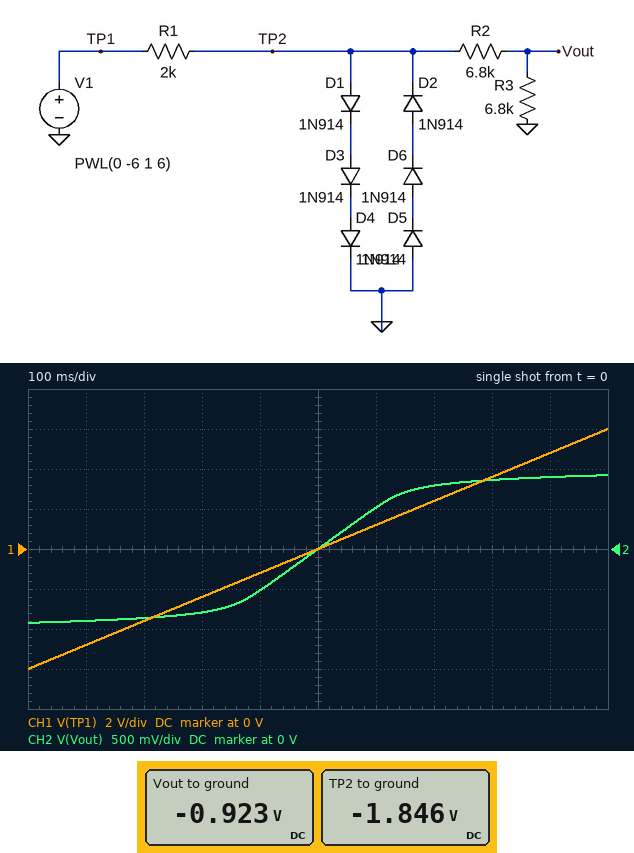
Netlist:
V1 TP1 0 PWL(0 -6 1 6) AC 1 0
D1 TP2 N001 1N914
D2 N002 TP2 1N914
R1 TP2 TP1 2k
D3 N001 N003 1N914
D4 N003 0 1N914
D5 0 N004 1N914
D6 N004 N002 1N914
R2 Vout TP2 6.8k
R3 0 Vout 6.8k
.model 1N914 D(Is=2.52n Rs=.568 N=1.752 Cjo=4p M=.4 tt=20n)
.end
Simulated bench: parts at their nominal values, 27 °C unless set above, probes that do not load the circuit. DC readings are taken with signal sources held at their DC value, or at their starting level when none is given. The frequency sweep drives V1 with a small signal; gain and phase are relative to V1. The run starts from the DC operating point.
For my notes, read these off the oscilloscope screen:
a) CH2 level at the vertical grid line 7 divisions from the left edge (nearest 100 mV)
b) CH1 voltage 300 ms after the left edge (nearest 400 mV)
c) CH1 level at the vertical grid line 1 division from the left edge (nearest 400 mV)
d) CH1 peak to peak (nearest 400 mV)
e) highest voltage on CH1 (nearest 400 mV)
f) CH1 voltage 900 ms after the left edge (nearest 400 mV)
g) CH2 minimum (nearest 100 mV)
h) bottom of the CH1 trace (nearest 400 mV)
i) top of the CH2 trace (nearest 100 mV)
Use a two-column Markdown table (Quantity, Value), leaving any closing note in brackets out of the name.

| Quantity | Value |
|---|---|
| CH2 level at the vertical grid line 7 divisions from the left edge | 800 mV |
| CH1 voltage 300 ms after the left edge | -2.4 V |
| CH1 level at the vertical grid line 1 division from the left edge | -4.8 V |
| CH1 peak to peak | 12.0 V |
| highest voltage on CH1 | 6.0 V |
| CH1 voltage 900 ms after the left edge | 4.8 V |
| CH2 minimum | -900 mV |
| bottom of the CH1 trace | -6.0 V |
| top of the CH2 trace | 900 mV |
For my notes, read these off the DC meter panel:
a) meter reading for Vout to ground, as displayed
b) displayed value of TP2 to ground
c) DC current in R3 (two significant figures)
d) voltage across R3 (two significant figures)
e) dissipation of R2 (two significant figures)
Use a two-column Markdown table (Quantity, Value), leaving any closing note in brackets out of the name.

| Quantity | Value |
|---|---|
| meter reading for Vout to ground, as displayed | -0.923 V |
| displayed value of TP2 to ground | -1.846 V |
| DC current in R3 | 140 µA |
| voltage across R3 | 920 mV |
| dissipation of R2 | 130 µW |
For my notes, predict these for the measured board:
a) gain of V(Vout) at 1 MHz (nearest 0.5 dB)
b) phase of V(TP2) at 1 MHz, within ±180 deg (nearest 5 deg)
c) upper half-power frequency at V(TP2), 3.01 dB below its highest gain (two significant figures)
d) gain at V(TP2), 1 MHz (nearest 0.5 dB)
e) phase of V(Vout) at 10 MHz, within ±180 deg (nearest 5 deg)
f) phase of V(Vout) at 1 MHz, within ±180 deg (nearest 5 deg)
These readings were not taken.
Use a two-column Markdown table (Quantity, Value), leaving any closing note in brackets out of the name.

| Quantity | Value |
|---|---|
| gain of V(Vout) at 1 MHz | -35.5 dB |
| phase of V(TP2) at 1 MHz, within ±180 deg | -5 deg |
| upper half-power frequency at V(TP2), 3.01 dB below its highest gain | 8.2 MHz |
| gain at V(TP2), 1 MHz | -29.5 dB |
| phase of V(Vout) at 10 MHz, within ±180 deg | -50 deg |
| phase of V(Vout) at 1 MHz, within ±180 deg | -5 deg |
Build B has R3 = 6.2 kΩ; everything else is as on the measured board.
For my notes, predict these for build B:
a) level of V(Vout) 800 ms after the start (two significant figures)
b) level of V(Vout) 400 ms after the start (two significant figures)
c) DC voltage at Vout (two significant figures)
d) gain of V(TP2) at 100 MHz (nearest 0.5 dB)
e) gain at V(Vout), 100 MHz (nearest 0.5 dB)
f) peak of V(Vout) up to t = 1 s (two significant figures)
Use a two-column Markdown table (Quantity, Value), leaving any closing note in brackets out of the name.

| Quantity | Value |
|---|---|
| level of V(Vout) 800 ms after the start | 820 mV |
| level of V(Vout) 400 ms after the start | -490 mV |
| DC voltage at Vout | -880 mV |
| gain of V(TP2) at 100 MHz | -50.5 dB |
| gain at V(Vout), 100 MHz | -57.0 dB |
| peak of V(Vout) up to t = 1 s | 880 mV |
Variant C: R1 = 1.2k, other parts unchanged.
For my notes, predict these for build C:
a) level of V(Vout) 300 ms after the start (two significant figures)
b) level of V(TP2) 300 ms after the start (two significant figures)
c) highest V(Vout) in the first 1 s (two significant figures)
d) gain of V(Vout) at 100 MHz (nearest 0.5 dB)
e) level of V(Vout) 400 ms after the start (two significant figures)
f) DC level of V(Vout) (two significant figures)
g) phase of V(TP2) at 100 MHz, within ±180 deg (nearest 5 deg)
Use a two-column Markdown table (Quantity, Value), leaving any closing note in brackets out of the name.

| Quantity | Value |
|---|---|
| level of V(Vout) 300 ms after the start | -830 mV |
| level of V(TP2) 300 ms after the start | -1.7 V |
| highest V(Vout) in the first 1 s | 960 mV |
| gain of V(Vout) at 100 MHz | -56.0 dB |
| level of V(Vout) 400 ms after the start | -550 mV |
| DC level of V(Vout) | -960 mV |
| phase of V(TP2) at 100 MHz, within ±180 deg | -60 deg |
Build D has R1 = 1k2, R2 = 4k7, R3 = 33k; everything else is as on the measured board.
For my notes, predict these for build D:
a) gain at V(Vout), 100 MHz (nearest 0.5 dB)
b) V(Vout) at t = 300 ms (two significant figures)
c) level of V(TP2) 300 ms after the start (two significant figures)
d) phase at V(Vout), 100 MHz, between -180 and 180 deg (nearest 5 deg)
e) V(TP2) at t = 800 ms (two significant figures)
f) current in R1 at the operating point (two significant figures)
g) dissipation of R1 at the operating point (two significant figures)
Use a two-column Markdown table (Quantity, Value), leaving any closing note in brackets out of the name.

| Quantity | Value |
|---|---|
| gain at V(Vout), 100 MHz | -51.5 dB |
| V(Vout) at t = 300 ms | -1.5 V |
| level of V(TP2) 300 ms after the start | -1.7 V |
| phase at V(Vout), 100 MHz, between -180 and 180 deg | -60 deg |
| V(TP2) at t = 800 ms | 1.8 V |
| current in R1 at the operating point | 3.4 mA |
| dissipation of R1 at the operating point | 14 mW |
